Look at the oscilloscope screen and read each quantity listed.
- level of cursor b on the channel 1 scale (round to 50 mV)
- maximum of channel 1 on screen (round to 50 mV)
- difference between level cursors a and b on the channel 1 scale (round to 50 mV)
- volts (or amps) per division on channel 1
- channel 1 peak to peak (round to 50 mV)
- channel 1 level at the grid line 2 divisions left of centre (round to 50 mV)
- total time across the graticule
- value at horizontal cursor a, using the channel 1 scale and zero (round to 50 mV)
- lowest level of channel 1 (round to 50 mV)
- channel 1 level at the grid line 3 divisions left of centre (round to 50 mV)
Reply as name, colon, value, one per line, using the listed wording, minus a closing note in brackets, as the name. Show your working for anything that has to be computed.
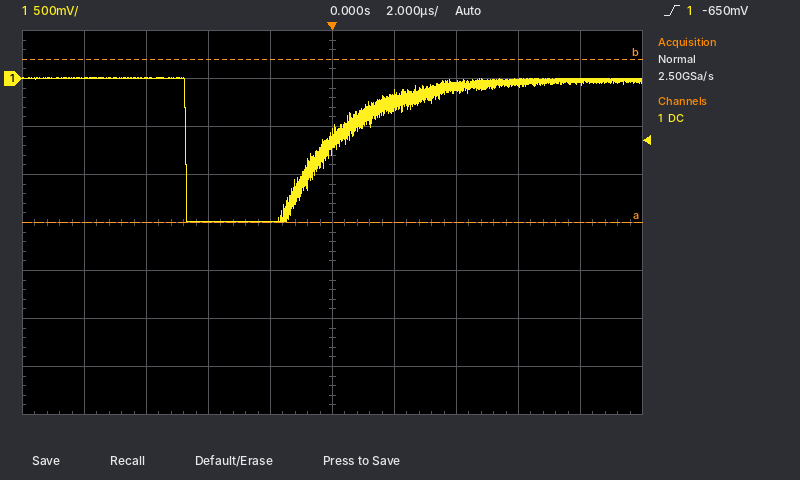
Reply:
level of cursor b on the channel 1 scale: 200 mV
maximum of channel 1 on screen: 0 mV
difference between level cursors a and b on the channel 1 scale: 1.70 V
volts (or amps) per division on channel 1: 500 mV
channel 1 peak to peak: 0 mV − (-1.50 V) = 1.50 V
channel 1 level at the grid line 2 divisions left of centre: -1.50 V
total time across the graticule: 20 µs
value at horizontal cursor a, using the channel 1 scale and zero: -1.50 V
lowest level of channel 1: -1.50 V
channel 1 level at the grid line 3 divisions left of centre: 0 mV
